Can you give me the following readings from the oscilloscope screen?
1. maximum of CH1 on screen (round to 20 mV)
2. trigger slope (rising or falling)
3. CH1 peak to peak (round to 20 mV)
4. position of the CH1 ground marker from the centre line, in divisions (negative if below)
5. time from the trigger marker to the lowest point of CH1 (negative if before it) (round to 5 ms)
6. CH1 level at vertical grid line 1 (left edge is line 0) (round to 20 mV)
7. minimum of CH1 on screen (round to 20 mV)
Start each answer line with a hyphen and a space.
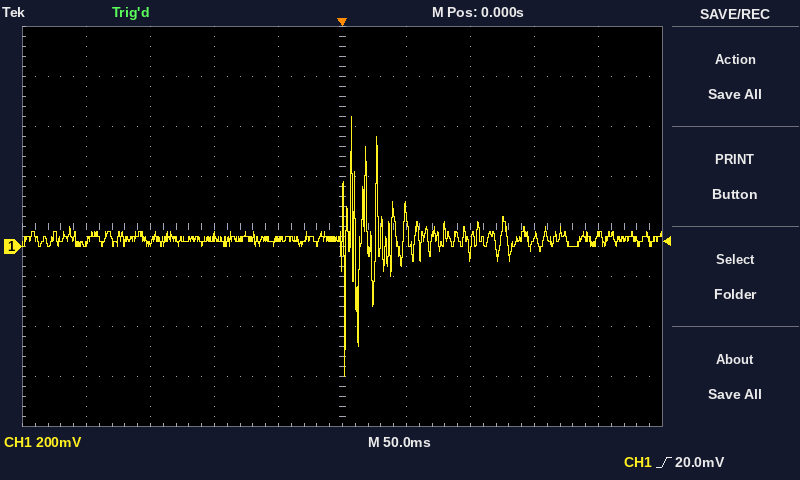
- 520 mV
- rising
- 1.04 V
- -0.4 div
- 0 ms
- 20 mV
- -520 mV
